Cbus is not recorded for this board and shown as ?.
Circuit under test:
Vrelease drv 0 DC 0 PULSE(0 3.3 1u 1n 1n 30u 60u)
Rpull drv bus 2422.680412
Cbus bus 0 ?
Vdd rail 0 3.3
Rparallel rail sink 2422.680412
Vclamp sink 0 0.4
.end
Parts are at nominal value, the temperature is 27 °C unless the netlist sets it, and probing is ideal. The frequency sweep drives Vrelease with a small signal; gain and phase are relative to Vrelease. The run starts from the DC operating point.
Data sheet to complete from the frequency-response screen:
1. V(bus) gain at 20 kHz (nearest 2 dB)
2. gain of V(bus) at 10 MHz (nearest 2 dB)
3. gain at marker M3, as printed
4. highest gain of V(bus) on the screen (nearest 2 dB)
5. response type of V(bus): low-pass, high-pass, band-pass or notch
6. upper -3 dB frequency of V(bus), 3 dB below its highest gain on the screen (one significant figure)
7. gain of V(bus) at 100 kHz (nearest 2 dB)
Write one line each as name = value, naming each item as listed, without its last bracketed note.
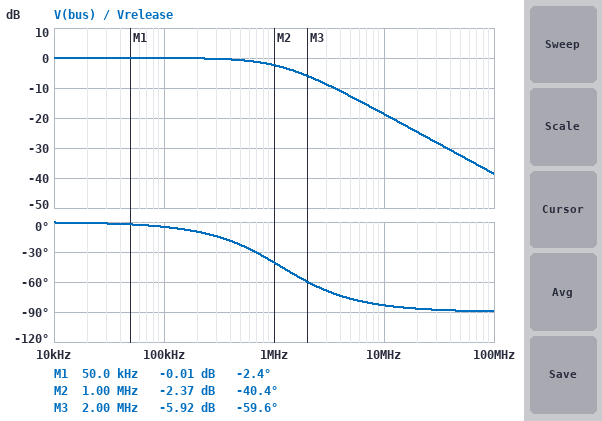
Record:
V(bus) gain at 20 kHz = 0 dB
gain of V(bus) at 10 MHz = -18 dB
gain at marker M3, as printed = -5.92 dB
highest gain of V(bus) on the screen = 0 dB
response type of V(bus): low-pass, high-pass, band-pass or notch = low-pass
upper -3 dB frequency of V(bus), 3 dB below its highest gain on the screen = 1 MHz
gain of V(bus) at 100 kHz = 0 dB
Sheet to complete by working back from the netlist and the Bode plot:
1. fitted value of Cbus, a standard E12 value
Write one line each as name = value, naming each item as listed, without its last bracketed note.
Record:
fitted value of Cbus, a standard E12 value = 56 pF
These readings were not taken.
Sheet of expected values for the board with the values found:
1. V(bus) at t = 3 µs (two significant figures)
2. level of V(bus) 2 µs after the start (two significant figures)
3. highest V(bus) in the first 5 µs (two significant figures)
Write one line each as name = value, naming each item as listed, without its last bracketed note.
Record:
V(bus) at t = 3 µs = 3.3 V
level of V(bus) 2 µs after the start = 3.3 V
highest V(bus) in the first 5 µs = 3.3 V
